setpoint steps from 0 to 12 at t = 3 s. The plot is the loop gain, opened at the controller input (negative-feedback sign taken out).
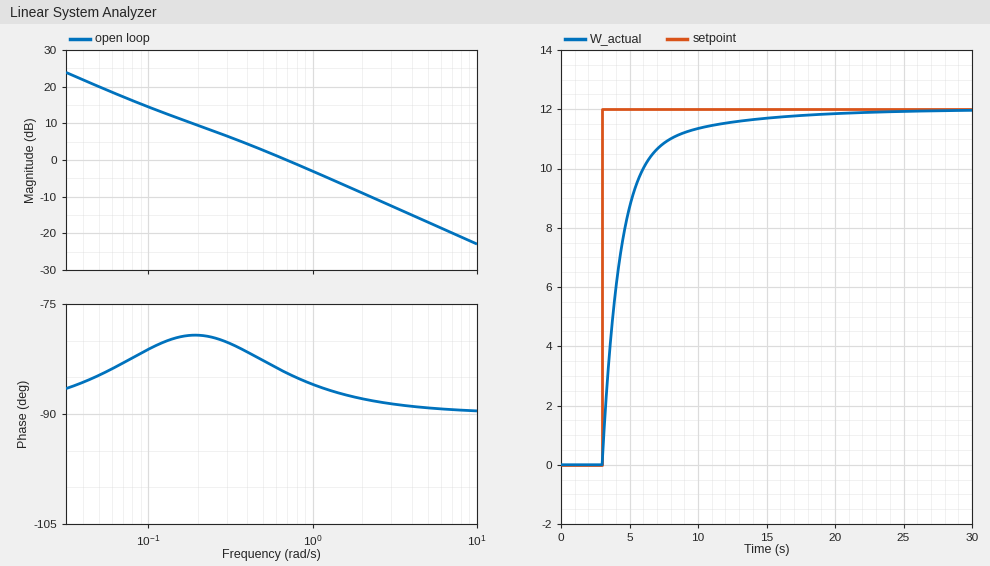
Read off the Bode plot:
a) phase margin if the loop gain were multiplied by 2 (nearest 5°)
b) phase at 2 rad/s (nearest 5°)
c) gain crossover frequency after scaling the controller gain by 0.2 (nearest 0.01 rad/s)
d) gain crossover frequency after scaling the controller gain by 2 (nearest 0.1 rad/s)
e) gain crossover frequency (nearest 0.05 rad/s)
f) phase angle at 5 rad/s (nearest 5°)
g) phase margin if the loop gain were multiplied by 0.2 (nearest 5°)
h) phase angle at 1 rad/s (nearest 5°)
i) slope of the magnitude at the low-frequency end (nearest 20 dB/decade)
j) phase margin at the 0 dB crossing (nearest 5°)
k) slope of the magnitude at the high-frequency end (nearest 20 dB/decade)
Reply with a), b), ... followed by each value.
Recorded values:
a) 95°
b) -90°
c) 0.11 rad/s
d) 1.4 rad/s
e) 0.70 rad/s
f) -90°
g) 100°
h) -85°
i) -20 dB/decade
j) 95°
k) -20 dB/decade
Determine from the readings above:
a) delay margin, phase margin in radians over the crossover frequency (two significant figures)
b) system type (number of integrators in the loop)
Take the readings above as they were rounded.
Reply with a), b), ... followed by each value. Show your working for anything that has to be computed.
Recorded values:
a) 95 × π / 180 / 0.7 = 2.4 s
b) 1
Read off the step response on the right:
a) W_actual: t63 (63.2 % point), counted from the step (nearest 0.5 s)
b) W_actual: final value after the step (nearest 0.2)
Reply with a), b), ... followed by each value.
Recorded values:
a) 1.5 s
b) 12.0
